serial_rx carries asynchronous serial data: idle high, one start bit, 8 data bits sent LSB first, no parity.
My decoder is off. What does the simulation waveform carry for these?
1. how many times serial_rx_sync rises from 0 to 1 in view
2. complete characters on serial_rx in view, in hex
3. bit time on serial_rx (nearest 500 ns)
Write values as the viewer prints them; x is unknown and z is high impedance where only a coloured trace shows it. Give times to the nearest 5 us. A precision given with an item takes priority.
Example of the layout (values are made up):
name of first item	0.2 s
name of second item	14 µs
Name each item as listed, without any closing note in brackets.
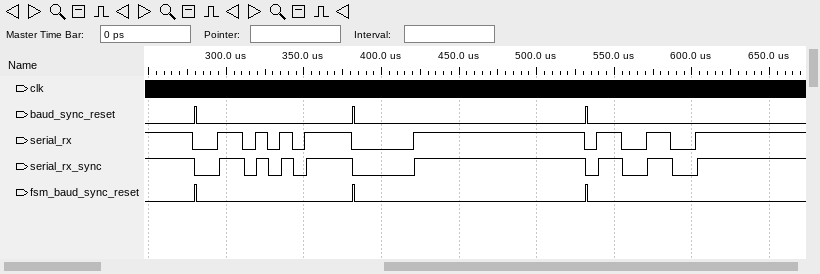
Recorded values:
how many times serial_rx_sync rises from 0 to 1 in view	8
complete characters on serial_rx in view, in hex	56, F0, 33
bit time on serial_rx	8000 ns
